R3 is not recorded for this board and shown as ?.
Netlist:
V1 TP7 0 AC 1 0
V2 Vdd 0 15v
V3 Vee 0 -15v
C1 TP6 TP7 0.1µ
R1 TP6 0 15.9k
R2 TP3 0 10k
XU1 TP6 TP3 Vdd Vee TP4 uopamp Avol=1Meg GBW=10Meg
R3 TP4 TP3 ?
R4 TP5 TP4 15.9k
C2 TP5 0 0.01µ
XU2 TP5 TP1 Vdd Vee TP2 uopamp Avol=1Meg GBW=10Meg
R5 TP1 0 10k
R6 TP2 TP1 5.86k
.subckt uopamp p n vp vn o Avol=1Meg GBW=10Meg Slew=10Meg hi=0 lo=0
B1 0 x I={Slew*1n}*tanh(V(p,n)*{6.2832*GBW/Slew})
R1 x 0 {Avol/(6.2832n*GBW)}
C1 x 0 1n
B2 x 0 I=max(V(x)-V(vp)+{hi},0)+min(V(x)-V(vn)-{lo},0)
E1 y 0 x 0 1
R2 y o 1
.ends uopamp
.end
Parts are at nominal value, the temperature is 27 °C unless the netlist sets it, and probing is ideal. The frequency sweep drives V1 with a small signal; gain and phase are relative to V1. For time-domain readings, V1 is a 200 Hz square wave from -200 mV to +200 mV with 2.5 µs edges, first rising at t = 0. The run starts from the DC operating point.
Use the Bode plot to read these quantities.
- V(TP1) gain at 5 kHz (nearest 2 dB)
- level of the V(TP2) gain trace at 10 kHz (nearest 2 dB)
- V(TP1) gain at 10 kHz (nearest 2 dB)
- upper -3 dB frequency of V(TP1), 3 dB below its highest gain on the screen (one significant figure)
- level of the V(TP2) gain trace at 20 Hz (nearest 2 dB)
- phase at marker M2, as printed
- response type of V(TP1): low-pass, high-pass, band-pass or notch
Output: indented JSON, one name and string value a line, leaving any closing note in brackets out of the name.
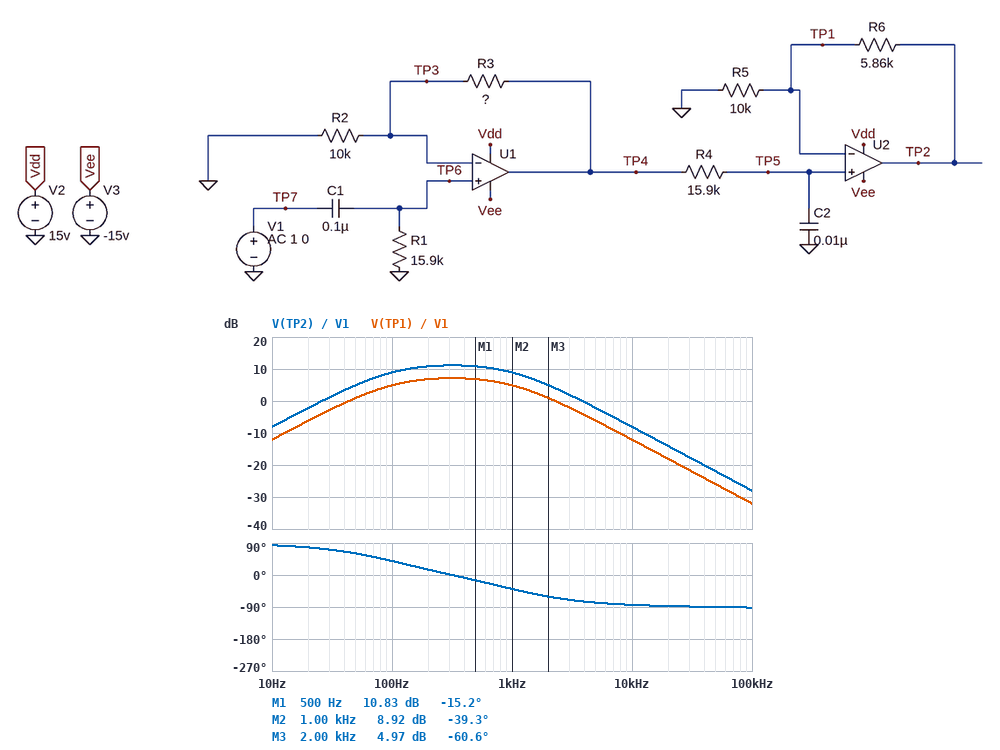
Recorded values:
{
  "V(TP1) gain at 5 kHz": "-6 dB",
  "level of the V(TP2) gain trace at 10 kHz": "-8 dB",
  "V(TP1) gain at 10 kHz": "-12 dB",
  "upper -3 dB frequency of V(TP1), 3 dB below its highest gain on the screen": "1 kHz",
  "level of the V(TP2) gain trace at 20 Hz": "-2 dB",
  "phase at marker M2, as printed": "-39.3 deg",
  "response type of V(TP1): low-pass, high-pass, band-pass or notch": "band-pass"
}
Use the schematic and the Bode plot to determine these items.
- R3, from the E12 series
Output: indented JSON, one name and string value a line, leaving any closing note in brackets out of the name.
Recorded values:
{
  "R3, from the E12 series": "15 kΩ"
}
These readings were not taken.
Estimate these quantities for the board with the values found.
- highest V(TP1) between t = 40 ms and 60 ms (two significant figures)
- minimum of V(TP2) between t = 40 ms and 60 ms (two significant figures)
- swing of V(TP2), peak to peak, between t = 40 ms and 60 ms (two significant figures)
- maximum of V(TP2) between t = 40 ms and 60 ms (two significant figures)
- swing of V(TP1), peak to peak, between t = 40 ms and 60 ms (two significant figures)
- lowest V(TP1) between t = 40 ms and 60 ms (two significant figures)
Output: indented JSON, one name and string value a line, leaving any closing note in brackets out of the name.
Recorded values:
{
  "highest V(TP1) between t = 40 ms and 60 ms": "630 mV",
  "minimum of V(TP2) between t = 40 ms and 60 ms": "-1.0 V",
  "swing of V(TP2), peak to peak, between t = 40 ms and 60 ms": "2.0 V",
  "maximum of V(TP2) between t = 40 ms and 60 ms": "1.0 V",
  "swing of V(TP1), peak to peak, between t = 40 ms and 60 ms": "1.3 V",
  "lowest V(TP1) between t = 40 ms and 60 ms": "-630 mV"
}
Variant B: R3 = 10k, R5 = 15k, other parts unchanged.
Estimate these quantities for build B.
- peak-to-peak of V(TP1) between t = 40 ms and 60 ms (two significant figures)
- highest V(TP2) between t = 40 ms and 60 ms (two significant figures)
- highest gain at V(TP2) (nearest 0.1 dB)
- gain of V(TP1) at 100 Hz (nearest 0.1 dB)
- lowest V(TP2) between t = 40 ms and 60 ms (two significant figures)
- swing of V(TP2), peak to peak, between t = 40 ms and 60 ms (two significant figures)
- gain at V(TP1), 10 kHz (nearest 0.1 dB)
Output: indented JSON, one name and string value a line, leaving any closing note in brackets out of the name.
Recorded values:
{
  "peak-to-peak of V(TP1) between t = 40 ms and 60 ms": "1.0 V",
  "highest V(TP2) between t = 40 ms and 60 ms": "700 mV",
  "highest gain at V(TP2)": "8.1 dB",
  "gain of V(TP1) at 100 Hz": "3.0 dB",
  "lowest V(TP2) between t = 40 ms and 60 ms": "-700 mV",
  "swing of V(TP2), peak to peak, between t = 40 ms and 60 ms": "1.4 V",
  "gain at V(TP1), 10 kHz": "-14.0 dB"
}
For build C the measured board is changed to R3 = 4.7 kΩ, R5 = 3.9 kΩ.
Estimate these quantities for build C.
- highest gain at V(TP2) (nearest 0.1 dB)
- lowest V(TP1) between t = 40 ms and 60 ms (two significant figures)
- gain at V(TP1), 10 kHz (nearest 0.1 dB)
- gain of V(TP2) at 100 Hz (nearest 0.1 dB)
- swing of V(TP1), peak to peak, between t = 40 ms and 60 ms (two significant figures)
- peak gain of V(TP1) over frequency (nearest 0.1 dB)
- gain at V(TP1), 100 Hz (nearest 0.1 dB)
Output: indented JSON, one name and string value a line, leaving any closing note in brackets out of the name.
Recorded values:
{
  "highest gain at V(TP2)": "10.5 dB",
  "lowest V(TP1) between t = 40 ms and 60 ms": "-370 mV",
  "gain at V(TP1), 10 kHz": "-16.7 dB",
  "gain of V(TP2) at 100 Hz": "8.3 dB",
  "swing of V(TP1), peak to peak, between t = 40 ms and 60 ms": "740 mV",
  "peak gain of V(TP1) over frequency": "2.5 dB",
  "gain at V(TP1), 100 Hz": "0.3 dB"
}
